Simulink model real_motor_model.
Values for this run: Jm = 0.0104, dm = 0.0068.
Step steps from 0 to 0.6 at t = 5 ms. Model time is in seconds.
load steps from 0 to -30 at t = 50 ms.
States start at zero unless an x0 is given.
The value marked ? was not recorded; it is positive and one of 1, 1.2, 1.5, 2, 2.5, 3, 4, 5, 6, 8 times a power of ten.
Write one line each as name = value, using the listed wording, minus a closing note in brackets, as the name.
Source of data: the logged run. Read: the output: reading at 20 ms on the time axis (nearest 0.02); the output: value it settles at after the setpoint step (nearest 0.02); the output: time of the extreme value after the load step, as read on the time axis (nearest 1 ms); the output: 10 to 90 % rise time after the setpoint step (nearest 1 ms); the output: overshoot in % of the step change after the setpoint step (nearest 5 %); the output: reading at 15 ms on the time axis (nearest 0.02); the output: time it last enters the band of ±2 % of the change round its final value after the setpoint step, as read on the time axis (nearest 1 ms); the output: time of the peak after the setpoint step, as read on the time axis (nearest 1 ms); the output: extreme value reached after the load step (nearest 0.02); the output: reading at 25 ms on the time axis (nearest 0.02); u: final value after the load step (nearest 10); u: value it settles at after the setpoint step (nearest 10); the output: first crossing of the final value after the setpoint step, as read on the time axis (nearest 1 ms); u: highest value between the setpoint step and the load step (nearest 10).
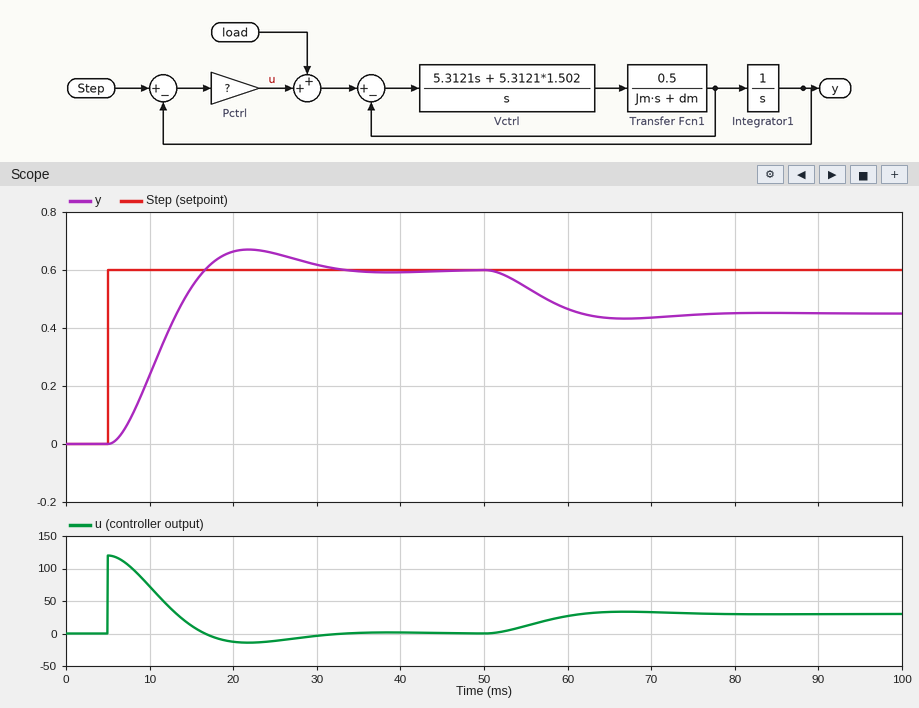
the output: reading at 20 ms on the time axis = 0.66
the output: value it settles at after the setpoint step = 0.60
the output: time of the extreme value after the load step, as read on the time axis = 67 ms
the output: 10 to 90 % rise time after the setpoint step = 8 ms
the output: overshoot in % of the step change after the setpoint step = 10 %
the output: reading at 15 ms on the time axis = 0.54
the output: time it last enters the band of ±2 % of the change round its final value after the setpoint step, as read on the time axis = 31 ms
the output: time of the peak after the setpoint step, as read on the time axis = 22 ms
the output: extreme value reached after the load step = 0.44
the output: reading at 25 ms on the time axis = 0.66
u: final value after the load step = 30
u: value it settles at after the setpoint step = 0
the output: first crossing of the final value after the setpoint step, as read on the time axis = 17 ms
u: highest value between the setpoint step and the load step = 120
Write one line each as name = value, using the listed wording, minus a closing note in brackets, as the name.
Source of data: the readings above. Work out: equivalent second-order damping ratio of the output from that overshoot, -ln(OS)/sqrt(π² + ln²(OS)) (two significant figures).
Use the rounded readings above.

equivalent second-order damping ratio of the output from that overshoot, -ln(OS)/sqrt(π² + ln²(OS)) = 0.59
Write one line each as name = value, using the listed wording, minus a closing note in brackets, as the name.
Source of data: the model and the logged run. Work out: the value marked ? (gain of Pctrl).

the value marked ? = 200
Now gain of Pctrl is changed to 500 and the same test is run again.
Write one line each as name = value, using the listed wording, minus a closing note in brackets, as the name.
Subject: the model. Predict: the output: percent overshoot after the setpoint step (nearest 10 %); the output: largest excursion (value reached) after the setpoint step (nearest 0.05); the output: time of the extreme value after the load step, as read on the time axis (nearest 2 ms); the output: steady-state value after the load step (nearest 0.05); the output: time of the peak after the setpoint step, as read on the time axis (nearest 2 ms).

the output: percent overshoot after the setpoint step = 30 %
the output: largest excursion (value reached) after the setpoint step = 0.80
the output: time of the extreme value after the load step, as read on the time axis = 60 ms
the output: steady-state value after the load step = 0.55
the output: time of the peak after the setpoint step, as read on the time axis = 14 ms
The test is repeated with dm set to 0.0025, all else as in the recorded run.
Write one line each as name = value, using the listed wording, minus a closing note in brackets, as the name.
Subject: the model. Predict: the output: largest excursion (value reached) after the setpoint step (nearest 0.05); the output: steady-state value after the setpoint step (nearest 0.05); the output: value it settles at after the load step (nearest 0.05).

the output: largest excursion (value reached) after the setpoint step = 0.65
the output: steady-state value after the setpoint step = 0.60
the output: value it settles at after the load step = 0.45
